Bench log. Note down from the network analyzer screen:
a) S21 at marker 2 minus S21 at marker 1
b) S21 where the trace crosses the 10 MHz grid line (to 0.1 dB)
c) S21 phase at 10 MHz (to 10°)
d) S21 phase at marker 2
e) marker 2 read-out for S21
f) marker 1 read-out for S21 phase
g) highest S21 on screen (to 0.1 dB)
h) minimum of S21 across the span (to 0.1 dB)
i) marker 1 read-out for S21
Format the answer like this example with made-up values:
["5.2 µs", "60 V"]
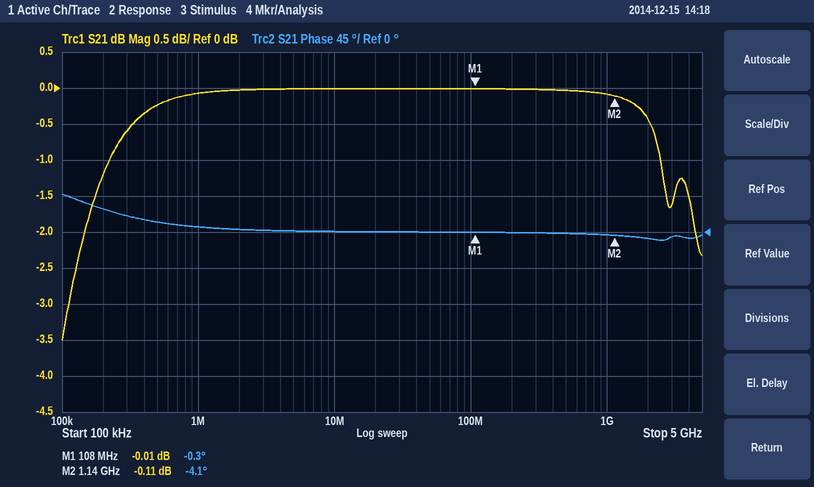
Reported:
["-0.10 dB", "0.0 dB", "0°", "-4.1°", "-0.11 dB", "-0.3°", "0.0 dB", "-3.5 dB", "-0.01 dB"]
